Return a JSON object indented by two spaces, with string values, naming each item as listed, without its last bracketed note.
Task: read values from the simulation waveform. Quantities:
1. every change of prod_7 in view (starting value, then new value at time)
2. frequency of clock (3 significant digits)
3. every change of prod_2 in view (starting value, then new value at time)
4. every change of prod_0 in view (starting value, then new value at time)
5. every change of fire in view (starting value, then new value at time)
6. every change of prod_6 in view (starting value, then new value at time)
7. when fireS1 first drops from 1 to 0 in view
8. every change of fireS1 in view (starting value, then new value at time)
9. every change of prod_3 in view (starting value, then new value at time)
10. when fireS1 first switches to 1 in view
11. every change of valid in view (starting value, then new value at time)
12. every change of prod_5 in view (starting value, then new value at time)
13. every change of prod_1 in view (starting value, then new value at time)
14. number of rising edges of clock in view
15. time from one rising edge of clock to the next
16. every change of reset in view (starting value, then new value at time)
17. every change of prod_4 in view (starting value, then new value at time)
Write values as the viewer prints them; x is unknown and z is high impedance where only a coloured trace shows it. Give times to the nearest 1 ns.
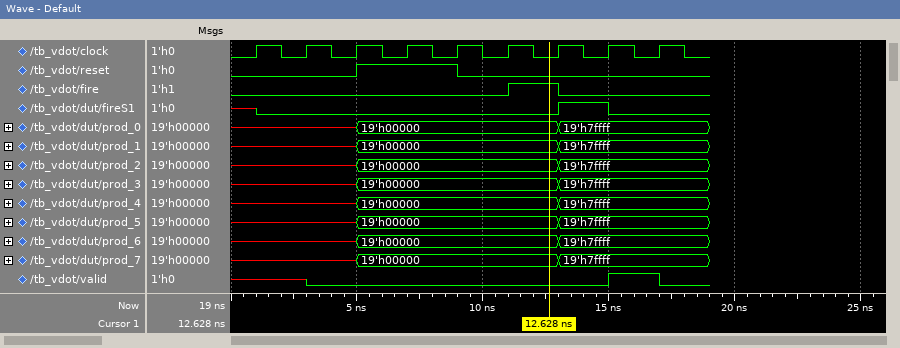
{
  "every change of prod_7 in view": "x, 19'h00000 at 5 ns, 19'h7ffff at 13 ns",
  "frequency of clock": "500 MHz",
  "every change of prod_2 in view": "x, 19'h00000 at 5 ns, 19'h7ffff at 13 ns",
  "every change of prod_0 in view": "x, 19'h00000 at 5 ns, 19'h7ffff at 13 ns",
  "every change of fire in view": "0, 1 at 11 ns, 0 at 13 ns",
  "every change of prod_6 in view": "x, 19'h00000 at 5 ns, 19'h7ffff at 13 ns",
  "when fireS1 first drops from 1 to 0 in view": "15 ns",
  "every change of fireS1 in view": "x, 0 at 1 ns, 1 at 13 ns, 0 at 15 ns",
  "every change of prod_3 in view": "x, 19'h00000 at 5 ns, 19'h7ffff at 13 ns",
  "when fireS1 first switches to 1 in view": "13 ns",
  "every change of valid in view": "x, 0 at 3 ns, 1 at 15 ns, 0 at 17 ns",
  "every change of prod_5 in view": "x, 19'h00000 at 5 ns, 19'h7ffff at 13 ns",
  "every change of prod_1 in view": "x, 19'h00000 at 5 ns, 19'h7ffff at 13 ns",
  "number of rising edges of clock in view": "9",
  "time from one rising edge of clock to the next": "2 ns",
  "every change of reset in view": "0, 1 at 5 ns, 0 at 9 ns",
  "every change of prod_4 in view": "x, 19'h00000 at 5 ns, 19'h7ffff at 13 ns"
}
